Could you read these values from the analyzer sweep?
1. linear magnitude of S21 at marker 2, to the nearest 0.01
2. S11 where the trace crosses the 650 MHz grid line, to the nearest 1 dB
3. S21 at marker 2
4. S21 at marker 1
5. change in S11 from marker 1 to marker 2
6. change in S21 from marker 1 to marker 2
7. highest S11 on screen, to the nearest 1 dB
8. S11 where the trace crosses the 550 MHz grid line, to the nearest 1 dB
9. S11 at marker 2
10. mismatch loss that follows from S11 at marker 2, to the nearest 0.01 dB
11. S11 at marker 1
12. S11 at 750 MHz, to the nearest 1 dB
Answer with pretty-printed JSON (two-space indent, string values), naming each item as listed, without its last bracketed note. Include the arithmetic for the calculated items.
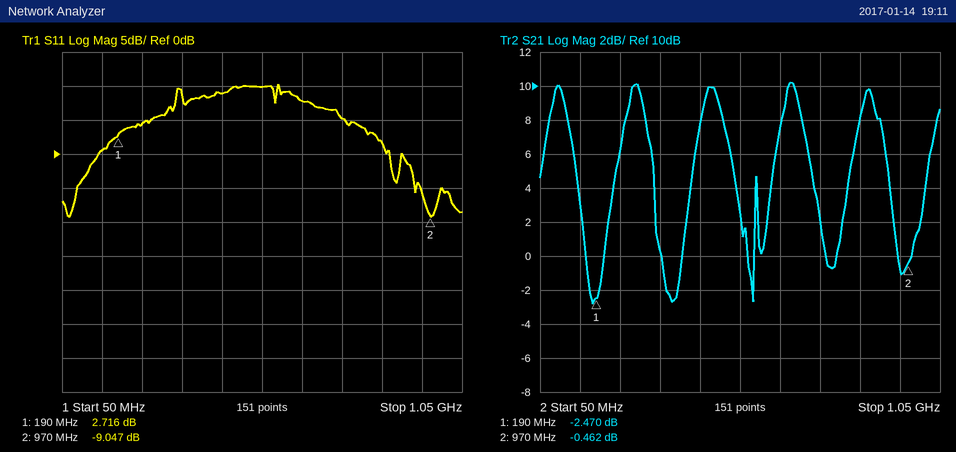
{
  "linear magnitude of S21 at marker 2, to the nearest 0.01": "10^(-0.462/20) ≈ 0.95",
  "S11 where the trace crosses the 650 MHz grid line, to the nearest 1 dB": "8 dB",
  "S21 at marker 2": "-0.462 dB",
  "S21 at marker 1": "-2.470 dB",
  "change in S11 from marker 1 to marker 2": "-9.047 − (2.716) = -11.763 dB",
  "change in S21 from marker 1 to marker 2": "-0.462 − (-2.47) = 2.008 dB",
  "highest S11 on screen, to the nearest 1 dB": "10 dB",
  "S11 where the trace crosses the 550 MHz grid line, to the nearest 1 dB": "10 dB",
  "S11 at marker 2": "-9.047 dB",
  "mismatch loss that follows from S11 at marker 2, to the nearest 0.01 dB": "−10 log10(1 − 10^(-9.047/10)) ≈ 0.58 dB",
  "S11 at marker 1": "2.716 dB",
  "S11 at 750 MHz, to the nearest 1 dB": "5 dB"
}
